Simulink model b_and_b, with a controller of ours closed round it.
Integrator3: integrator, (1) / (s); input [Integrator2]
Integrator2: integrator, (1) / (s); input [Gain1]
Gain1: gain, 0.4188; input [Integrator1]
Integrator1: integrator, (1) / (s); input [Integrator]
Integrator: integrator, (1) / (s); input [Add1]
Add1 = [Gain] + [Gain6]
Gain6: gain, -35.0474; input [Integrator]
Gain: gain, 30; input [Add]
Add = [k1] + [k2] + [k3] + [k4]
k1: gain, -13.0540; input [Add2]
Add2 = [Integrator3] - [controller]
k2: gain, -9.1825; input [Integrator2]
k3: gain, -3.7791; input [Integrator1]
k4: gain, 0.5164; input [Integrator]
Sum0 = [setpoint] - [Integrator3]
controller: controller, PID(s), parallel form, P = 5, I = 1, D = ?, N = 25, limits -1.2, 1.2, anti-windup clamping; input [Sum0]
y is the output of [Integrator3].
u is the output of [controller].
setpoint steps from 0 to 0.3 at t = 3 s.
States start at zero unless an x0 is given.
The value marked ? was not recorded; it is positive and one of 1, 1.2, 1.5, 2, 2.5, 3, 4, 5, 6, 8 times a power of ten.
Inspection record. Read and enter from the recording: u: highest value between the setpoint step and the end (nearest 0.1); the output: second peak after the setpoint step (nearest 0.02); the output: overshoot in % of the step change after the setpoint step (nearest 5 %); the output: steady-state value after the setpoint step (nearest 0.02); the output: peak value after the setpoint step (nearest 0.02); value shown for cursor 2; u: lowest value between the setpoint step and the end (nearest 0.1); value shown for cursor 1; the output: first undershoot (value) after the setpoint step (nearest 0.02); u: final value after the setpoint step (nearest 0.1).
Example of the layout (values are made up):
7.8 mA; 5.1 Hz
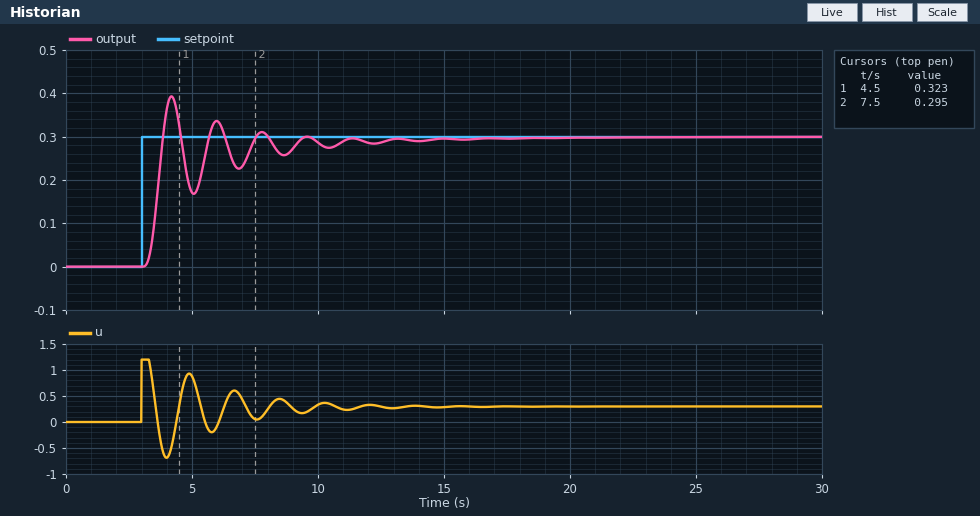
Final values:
1.2; 0.34; 30 %; 0.30; 0.40; 0.295; -0.7; 0.323; 0.16; 0.3
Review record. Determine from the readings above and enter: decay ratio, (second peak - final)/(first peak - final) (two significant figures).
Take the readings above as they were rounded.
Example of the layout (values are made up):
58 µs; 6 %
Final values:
0.40
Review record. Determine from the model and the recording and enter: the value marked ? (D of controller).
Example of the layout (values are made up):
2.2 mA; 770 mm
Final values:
1.2
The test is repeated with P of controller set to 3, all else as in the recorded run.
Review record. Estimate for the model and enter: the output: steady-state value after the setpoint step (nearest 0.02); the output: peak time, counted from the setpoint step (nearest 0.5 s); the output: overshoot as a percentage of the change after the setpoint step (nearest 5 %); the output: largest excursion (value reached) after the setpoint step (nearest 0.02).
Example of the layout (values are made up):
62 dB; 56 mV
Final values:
0.30; 1.5 s; 10 %; 0.32
